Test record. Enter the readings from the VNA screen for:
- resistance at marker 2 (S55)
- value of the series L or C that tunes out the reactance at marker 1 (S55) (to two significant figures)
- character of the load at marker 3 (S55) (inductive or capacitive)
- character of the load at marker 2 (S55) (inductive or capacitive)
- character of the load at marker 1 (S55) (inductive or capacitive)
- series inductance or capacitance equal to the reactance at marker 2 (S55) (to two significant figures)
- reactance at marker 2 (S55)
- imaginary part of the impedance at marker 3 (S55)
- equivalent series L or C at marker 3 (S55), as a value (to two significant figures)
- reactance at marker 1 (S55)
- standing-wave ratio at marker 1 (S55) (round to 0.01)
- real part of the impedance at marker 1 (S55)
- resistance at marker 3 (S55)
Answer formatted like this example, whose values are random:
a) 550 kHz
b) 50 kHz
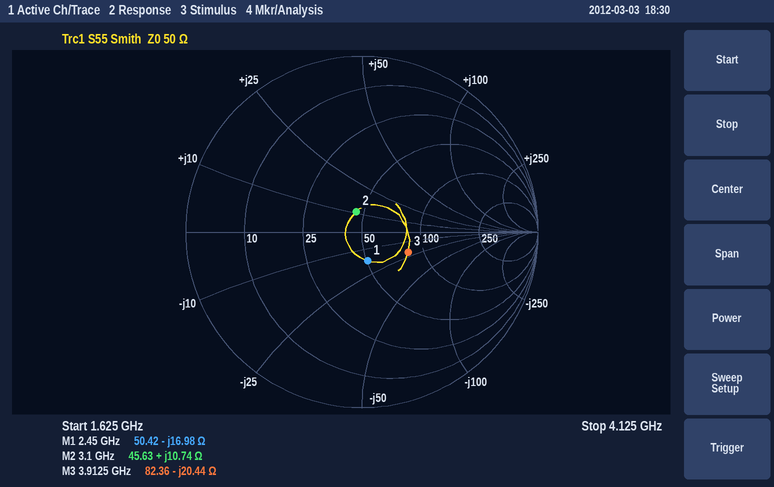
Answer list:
a) 45.63 Ω
b) 1.1 nH
c) capacitive
d) inductive
e) capacitive
f) 550 pH
g) +10.74 Ω
h) -20.44 Ω
i) 2.0 pF
j) -16.98 Ω
k) 1.40
l) 50.42 Ω
m) 82.36 Ω
